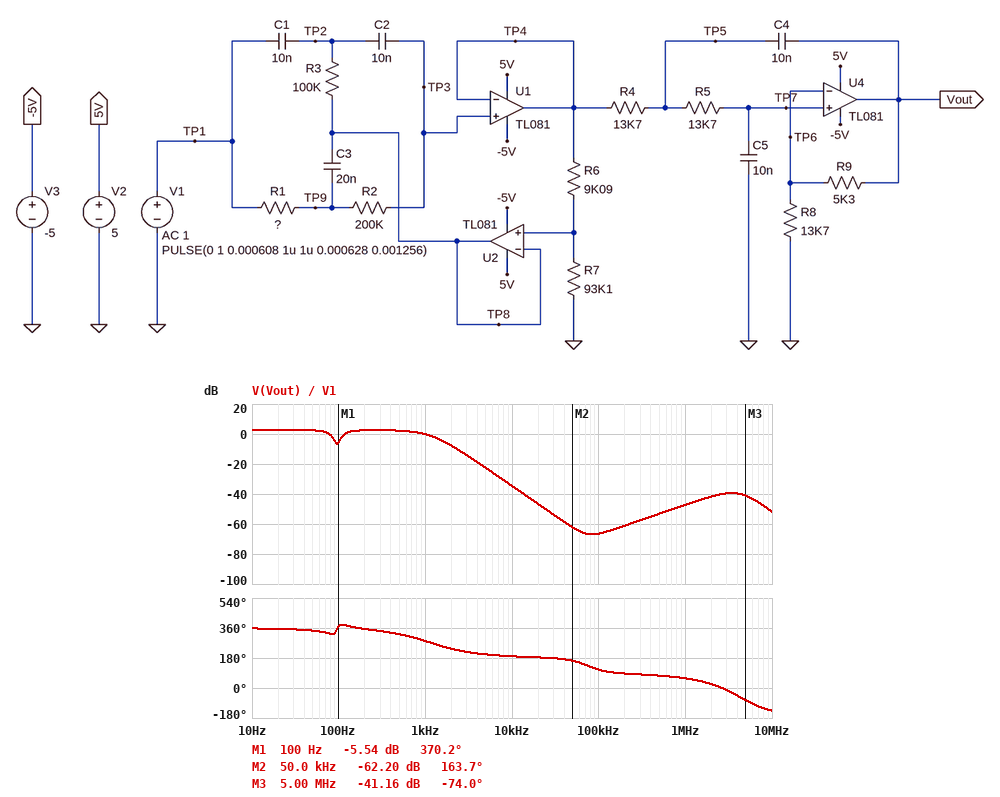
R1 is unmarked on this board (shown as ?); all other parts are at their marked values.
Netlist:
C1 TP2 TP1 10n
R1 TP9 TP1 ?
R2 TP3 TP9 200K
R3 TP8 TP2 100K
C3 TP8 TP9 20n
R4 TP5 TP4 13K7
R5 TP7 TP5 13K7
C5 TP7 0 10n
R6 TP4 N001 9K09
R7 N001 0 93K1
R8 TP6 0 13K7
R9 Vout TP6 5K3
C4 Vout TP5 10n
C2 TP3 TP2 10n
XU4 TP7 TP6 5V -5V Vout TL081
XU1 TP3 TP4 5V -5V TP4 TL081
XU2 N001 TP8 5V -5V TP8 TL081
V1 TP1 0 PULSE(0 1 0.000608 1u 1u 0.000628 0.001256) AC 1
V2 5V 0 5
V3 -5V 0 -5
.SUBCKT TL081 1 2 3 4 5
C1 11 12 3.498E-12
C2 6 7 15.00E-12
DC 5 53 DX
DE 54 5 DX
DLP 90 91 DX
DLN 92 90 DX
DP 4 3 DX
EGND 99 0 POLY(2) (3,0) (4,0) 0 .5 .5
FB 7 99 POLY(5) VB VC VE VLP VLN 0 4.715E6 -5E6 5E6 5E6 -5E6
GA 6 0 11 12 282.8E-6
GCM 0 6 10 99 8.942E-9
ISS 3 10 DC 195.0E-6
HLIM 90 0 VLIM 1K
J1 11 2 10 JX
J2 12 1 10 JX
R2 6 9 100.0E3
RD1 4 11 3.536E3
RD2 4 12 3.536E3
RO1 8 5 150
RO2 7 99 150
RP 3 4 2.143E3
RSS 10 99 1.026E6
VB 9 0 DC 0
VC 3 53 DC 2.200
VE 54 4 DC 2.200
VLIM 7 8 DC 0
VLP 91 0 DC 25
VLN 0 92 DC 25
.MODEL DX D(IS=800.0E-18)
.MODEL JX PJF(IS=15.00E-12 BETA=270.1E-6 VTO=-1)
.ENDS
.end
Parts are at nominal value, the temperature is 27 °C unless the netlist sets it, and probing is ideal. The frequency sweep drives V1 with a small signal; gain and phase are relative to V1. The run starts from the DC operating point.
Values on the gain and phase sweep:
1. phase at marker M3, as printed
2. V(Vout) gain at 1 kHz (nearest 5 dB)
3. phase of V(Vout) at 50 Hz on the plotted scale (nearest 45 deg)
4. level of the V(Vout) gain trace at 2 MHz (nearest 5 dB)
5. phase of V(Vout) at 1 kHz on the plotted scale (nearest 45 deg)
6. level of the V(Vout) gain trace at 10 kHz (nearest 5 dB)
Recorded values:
-74.0 deg
0 dB
360 deg
-40 dB
270 deg
-35 dB
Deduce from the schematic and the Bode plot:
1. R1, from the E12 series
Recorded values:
120 kΩ
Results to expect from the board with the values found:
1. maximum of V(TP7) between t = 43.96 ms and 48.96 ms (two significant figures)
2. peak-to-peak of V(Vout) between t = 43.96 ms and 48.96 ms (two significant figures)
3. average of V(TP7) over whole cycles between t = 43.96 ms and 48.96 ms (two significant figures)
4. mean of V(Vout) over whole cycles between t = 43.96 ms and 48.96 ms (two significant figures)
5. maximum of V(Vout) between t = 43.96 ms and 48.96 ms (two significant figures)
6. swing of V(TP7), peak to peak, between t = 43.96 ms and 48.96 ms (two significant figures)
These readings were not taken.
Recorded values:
1.0 V
1.4 V
500 mV
690 mV
1.4 V
1.0 V
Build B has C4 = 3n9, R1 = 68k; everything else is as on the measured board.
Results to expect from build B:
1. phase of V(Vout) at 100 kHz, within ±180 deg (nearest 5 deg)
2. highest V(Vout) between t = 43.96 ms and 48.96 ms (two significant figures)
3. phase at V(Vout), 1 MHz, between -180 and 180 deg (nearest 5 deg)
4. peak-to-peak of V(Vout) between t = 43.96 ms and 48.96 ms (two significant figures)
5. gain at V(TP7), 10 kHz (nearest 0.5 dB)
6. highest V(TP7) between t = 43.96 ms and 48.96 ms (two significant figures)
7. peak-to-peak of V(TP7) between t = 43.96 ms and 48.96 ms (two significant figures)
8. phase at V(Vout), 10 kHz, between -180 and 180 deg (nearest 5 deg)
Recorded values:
135 deg
1.3 V
60 deg
1.2 V
-30.0 dB
930 mV
850 mV
-150 deg
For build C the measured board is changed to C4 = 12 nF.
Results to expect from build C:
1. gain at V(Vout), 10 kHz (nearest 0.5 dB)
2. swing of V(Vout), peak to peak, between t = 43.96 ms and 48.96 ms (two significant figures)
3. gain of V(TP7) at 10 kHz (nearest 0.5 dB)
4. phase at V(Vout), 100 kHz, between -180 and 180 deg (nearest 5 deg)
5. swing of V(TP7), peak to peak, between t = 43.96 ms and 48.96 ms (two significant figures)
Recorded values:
-36.0 dB
1.5 V
-39.0 dB
105 deg
1.1 V
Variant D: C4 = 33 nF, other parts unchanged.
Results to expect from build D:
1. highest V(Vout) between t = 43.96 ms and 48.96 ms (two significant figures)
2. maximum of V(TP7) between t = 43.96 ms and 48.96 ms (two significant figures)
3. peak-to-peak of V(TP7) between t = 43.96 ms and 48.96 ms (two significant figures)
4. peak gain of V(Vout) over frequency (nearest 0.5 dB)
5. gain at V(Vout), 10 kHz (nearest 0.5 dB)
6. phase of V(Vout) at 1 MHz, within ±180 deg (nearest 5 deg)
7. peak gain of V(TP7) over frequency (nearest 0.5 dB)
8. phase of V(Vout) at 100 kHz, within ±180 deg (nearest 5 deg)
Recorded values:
1.9 V
1.4 V
1.7 V
11.0 dB
-45.0 dB
60 deg
8.0 dB
95 deg
